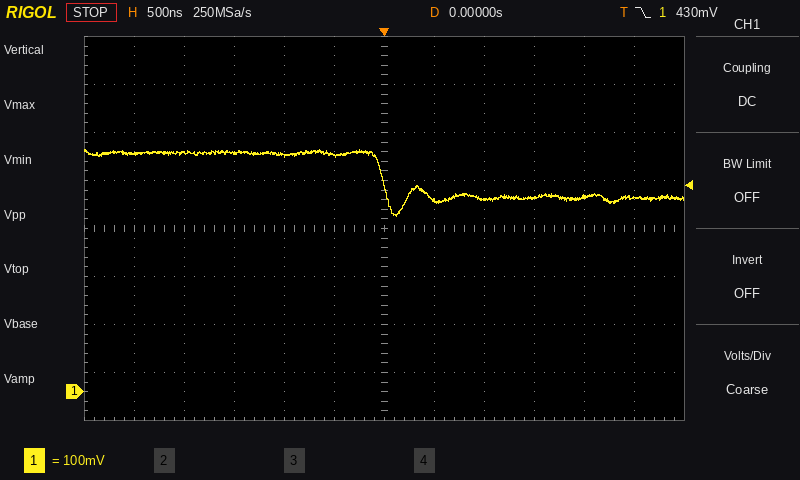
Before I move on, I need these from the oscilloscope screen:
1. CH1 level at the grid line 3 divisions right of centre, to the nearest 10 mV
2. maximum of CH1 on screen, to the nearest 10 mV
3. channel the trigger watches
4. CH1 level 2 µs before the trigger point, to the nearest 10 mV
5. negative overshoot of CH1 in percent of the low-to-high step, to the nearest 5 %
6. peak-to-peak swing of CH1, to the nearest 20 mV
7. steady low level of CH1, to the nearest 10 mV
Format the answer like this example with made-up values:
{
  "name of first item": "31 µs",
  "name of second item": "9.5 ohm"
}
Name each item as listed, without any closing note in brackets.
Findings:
{
  "CH1 level at the grid line 3 divisions right of centre, to the nearest 10 mV": "400 mV",
  "maximum of CH1 on screen, to the nearest 10 mV": "500 mV",
  "channel the trigger watches": "CH1",
  "CH1 level 2 µs before the trigger point, to the nearest 10 mV": "500 mV",
  "negative overshoot of CH1 in percent of the low-to-high step, to the nearest 5 %": "40 %",
  "peak-to-peak swing of CH1, to the nearest 20 mV": "140 mV",
  "steady low level of CH1, to the nearest 10 mV": "400 mV"
}
